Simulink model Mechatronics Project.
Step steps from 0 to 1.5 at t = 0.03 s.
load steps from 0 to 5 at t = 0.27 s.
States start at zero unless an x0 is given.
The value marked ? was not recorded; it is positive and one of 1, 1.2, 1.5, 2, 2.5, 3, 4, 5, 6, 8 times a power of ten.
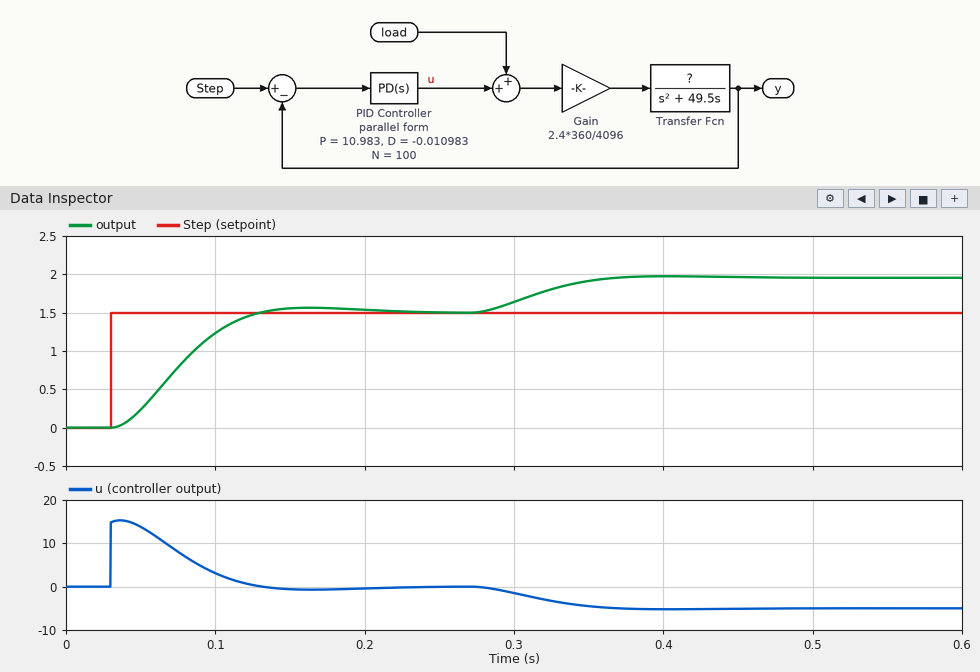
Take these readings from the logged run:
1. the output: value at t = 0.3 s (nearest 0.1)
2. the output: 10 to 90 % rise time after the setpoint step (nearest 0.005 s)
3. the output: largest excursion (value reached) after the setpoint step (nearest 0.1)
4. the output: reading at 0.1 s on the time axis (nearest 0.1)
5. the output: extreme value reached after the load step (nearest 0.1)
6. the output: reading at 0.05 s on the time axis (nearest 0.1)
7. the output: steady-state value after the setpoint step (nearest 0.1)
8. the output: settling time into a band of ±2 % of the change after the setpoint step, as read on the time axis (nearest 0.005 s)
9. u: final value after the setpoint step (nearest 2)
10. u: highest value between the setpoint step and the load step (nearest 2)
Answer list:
1.6
0.065 s
1.6
1.2
2.0
0.2
1.5
0.210 s
0
16
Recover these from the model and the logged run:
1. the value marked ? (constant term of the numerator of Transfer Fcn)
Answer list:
500
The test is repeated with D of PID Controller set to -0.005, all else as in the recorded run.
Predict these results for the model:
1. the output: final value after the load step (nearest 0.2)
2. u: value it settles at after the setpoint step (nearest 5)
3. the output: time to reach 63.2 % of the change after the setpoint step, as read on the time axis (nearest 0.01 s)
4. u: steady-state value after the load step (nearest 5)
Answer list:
2.0
0
0.08 s
-5
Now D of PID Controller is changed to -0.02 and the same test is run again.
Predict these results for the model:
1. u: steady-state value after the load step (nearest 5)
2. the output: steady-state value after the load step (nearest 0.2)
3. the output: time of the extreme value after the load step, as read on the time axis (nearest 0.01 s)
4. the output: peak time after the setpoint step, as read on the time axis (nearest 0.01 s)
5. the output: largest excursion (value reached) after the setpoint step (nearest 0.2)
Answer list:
-5
2.0
0.40 s
0.16 s
1.6
